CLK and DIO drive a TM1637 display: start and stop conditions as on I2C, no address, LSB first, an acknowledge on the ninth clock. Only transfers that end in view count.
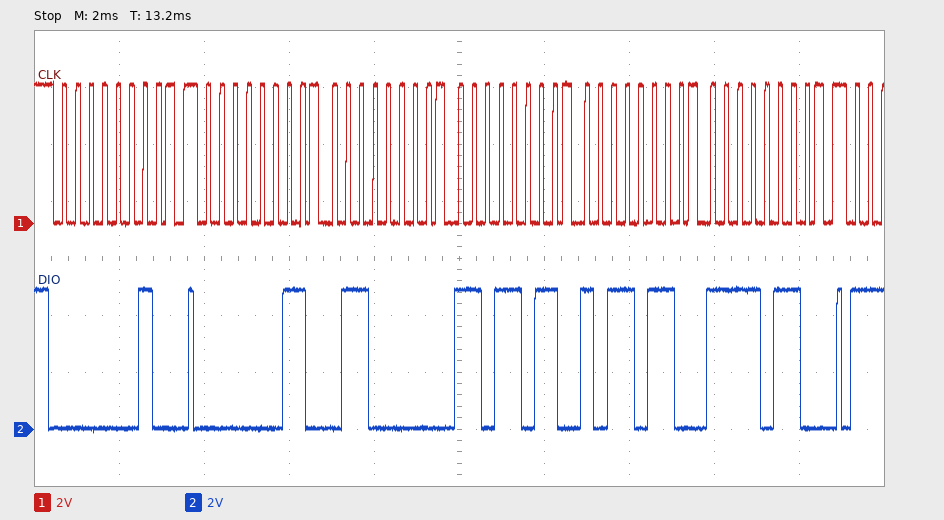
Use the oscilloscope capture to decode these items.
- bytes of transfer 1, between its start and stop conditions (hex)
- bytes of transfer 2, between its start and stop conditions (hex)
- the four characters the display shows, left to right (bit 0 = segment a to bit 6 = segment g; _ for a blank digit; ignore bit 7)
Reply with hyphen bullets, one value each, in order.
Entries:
- 40
- C0 06 DB 6D 6F
- 1259
